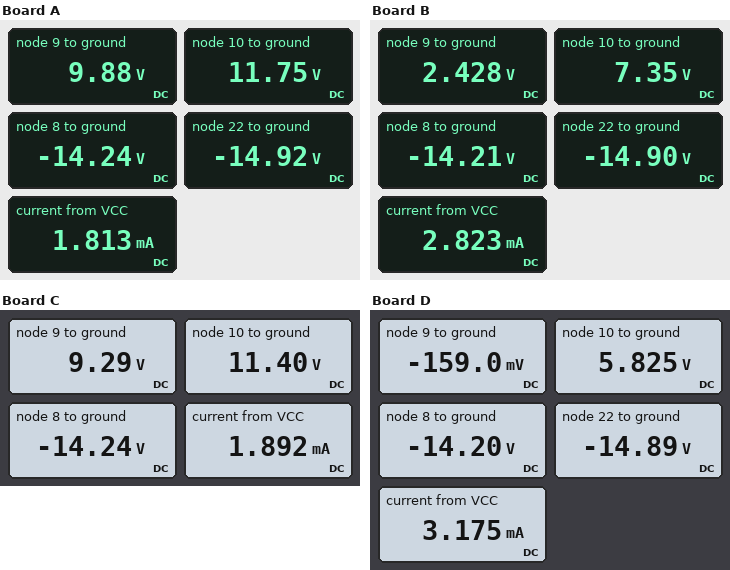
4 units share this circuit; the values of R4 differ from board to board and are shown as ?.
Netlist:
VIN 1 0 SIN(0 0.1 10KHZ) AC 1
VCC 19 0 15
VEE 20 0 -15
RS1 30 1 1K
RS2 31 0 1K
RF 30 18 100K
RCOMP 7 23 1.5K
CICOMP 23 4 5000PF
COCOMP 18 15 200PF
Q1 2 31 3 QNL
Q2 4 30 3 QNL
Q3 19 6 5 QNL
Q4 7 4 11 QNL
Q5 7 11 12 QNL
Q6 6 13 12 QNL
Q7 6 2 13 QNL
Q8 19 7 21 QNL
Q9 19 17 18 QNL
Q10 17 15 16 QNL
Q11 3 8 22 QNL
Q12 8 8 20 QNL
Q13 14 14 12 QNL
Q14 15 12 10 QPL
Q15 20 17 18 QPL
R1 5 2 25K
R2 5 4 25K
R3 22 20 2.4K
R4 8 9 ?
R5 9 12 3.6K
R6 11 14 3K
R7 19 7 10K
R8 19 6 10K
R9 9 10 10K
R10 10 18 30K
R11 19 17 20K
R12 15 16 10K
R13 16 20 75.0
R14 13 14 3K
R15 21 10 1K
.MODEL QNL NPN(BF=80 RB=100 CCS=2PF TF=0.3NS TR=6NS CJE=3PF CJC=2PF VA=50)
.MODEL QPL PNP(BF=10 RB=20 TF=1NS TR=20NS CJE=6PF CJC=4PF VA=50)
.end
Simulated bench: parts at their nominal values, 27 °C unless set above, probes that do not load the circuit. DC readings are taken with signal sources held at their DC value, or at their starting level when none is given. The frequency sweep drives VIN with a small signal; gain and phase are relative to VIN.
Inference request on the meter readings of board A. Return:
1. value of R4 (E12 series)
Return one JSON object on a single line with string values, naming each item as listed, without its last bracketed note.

{"value of R4": "47 kΩ"}
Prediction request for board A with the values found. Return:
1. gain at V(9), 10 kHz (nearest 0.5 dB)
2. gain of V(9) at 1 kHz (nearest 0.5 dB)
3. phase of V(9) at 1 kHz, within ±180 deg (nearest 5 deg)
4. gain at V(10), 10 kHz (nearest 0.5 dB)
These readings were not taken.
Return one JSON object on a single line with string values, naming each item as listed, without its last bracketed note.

{"gain at V(9), 10 kHz": "1.0 dB", "gain of V(9) at 1 kHz": "4.5 dB", "phase of V(9) at 1 kHz, within ±180 deg": "165 deg", "gain at V(10), 10 kHz": "2.0 dB"}
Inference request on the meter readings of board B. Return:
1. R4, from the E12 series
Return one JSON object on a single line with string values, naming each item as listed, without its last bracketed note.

{"R4, from the E12 series": "10 kΩ"}
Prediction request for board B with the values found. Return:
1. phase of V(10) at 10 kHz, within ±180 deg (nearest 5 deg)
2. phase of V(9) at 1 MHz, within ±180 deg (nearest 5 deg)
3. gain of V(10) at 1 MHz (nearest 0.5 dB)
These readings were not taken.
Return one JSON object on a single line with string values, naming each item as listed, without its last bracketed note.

{"phase of V(10) at 10 kHz, within ±180 deg": "80 deg", "phase of V(9) at 1 MHz, within ±180 deg": "10 deg", "gain of V(10) at 1 MHz": "3.5 dB"}
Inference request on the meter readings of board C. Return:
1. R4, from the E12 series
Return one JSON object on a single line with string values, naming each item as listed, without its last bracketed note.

{"R4, from the E12 series": "39 kΩ"}
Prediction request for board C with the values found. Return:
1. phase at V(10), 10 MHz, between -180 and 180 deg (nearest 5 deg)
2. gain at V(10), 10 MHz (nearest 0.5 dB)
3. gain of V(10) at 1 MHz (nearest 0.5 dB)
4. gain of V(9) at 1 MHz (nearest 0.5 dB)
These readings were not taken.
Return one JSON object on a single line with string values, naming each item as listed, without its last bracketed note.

{"phase at V(10), 10 MHz, between -180 and 180 deg": "-140 deg", "gain at V(10), 10 MHz": "-7.5 dB", "gain of V(10) at 1 MHz": "3.0 dB", "gain of V(9) at 1 MHz": "1.5 dB"}
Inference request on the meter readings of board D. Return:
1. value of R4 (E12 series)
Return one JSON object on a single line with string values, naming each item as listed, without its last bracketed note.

{"value of R4": "6.8 kΩ"}
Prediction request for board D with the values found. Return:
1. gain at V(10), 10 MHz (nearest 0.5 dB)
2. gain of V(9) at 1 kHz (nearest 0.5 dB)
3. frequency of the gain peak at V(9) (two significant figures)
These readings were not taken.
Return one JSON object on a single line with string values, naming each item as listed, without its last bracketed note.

{"gain at V(10), 10 MHz": "-3.5 dB", "gain of V(9) at 1 kHz": "-0.5 dB", "frequency of the gain peak at V(9)": "2.4 MHz"}
